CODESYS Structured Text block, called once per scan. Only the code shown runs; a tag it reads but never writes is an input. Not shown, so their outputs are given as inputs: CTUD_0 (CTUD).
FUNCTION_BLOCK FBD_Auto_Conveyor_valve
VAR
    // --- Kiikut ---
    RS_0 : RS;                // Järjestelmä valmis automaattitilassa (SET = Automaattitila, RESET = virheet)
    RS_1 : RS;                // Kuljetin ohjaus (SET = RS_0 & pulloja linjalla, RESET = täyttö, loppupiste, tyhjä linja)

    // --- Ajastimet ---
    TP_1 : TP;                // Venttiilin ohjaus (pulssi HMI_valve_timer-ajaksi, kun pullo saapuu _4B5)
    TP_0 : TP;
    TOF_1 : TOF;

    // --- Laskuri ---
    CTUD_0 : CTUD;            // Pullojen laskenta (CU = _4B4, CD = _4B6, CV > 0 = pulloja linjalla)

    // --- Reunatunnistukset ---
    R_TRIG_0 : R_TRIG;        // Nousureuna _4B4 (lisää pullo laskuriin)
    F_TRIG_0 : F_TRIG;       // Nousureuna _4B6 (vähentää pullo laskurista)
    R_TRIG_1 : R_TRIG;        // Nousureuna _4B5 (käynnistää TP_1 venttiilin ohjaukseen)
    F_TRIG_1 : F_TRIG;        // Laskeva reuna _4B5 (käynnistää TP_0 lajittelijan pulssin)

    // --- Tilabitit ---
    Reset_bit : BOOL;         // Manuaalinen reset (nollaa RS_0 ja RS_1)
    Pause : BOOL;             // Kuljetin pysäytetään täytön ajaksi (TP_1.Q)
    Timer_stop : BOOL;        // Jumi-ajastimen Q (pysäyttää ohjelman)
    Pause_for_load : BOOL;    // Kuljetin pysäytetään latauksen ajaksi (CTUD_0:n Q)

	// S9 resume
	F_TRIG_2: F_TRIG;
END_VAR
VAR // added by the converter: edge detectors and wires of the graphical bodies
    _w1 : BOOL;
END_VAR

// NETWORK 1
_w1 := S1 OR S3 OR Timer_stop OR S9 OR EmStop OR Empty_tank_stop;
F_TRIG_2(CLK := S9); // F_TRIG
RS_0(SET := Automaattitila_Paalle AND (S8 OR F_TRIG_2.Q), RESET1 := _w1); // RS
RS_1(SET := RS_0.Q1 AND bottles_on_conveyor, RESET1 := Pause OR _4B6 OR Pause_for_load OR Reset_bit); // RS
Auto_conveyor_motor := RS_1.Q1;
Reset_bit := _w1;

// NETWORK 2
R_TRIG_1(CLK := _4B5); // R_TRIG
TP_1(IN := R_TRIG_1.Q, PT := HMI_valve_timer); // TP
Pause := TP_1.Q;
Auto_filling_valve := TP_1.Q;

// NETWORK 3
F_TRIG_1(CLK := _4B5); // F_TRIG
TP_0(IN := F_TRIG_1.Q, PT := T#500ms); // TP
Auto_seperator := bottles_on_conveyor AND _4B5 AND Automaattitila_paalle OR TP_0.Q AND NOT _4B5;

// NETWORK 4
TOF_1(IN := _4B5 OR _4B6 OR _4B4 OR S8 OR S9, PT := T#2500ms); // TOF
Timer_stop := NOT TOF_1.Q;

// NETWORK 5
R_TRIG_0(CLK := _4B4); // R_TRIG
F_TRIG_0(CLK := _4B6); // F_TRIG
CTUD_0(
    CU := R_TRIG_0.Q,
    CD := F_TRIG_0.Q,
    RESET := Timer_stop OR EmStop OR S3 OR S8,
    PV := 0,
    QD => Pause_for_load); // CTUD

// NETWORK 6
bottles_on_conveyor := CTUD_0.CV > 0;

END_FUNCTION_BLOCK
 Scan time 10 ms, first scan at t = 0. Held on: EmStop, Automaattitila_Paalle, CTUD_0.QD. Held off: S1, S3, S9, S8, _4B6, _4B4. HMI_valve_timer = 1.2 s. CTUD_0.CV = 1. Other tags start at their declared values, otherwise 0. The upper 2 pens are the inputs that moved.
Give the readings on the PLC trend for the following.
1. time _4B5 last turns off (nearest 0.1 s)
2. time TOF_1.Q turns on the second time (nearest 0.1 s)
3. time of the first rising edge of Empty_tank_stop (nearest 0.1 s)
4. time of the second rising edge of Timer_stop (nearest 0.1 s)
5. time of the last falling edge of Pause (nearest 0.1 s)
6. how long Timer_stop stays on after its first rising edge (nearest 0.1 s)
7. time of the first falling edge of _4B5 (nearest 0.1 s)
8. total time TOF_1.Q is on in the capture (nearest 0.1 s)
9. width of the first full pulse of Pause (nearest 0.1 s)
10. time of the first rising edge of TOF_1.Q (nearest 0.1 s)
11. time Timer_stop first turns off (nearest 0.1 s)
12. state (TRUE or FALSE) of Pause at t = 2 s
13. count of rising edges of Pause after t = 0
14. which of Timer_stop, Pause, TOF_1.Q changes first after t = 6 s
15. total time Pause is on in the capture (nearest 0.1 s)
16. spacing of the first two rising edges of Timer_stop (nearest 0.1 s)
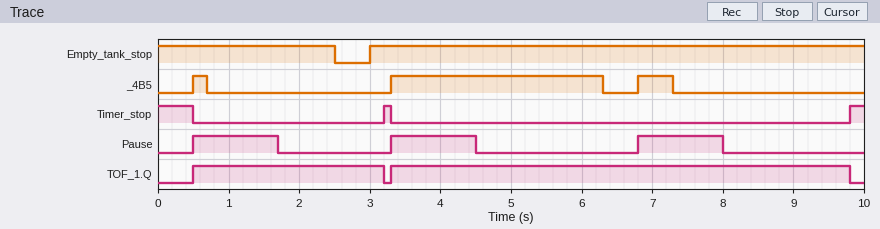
7.3 s
3.3 s
3.0 s
9.8 s
8.0 s
0.1 s
0.7 s
9.2 s
1.2 s
0.5 s
0.5 s
FALSE
3
Pause
3.6 s
6.6 s
